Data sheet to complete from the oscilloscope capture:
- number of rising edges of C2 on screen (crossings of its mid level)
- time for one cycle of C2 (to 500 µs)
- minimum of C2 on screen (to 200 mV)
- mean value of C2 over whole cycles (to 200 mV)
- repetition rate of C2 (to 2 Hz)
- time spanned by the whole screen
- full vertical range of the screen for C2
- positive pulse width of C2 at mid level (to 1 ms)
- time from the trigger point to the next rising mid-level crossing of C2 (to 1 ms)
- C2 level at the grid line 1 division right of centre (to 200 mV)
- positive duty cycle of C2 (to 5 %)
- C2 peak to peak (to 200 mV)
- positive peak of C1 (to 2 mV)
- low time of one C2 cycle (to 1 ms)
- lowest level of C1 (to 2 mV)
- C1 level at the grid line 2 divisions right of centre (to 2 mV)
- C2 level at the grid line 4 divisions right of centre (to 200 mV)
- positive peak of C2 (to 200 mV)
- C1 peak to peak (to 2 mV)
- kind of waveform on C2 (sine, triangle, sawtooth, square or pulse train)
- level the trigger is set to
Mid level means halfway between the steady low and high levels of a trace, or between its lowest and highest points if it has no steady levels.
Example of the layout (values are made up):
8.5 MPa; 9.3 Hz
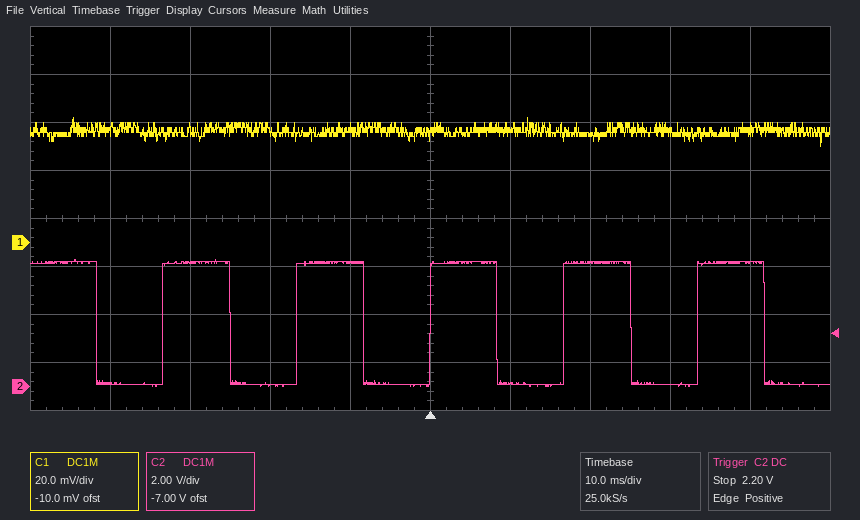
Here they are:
5; 16.5 ms; 0.0 V; 2.6 V; 60 Hz; 100 ms; 16 V; 8 ms; 17 ms; 200 mV; 50 %; 5.2 V; 52 mV; 8 ms; 40 mV; 44 mV; 5.2 V; 5.2 V; 12 mV; square; 2.20 V
